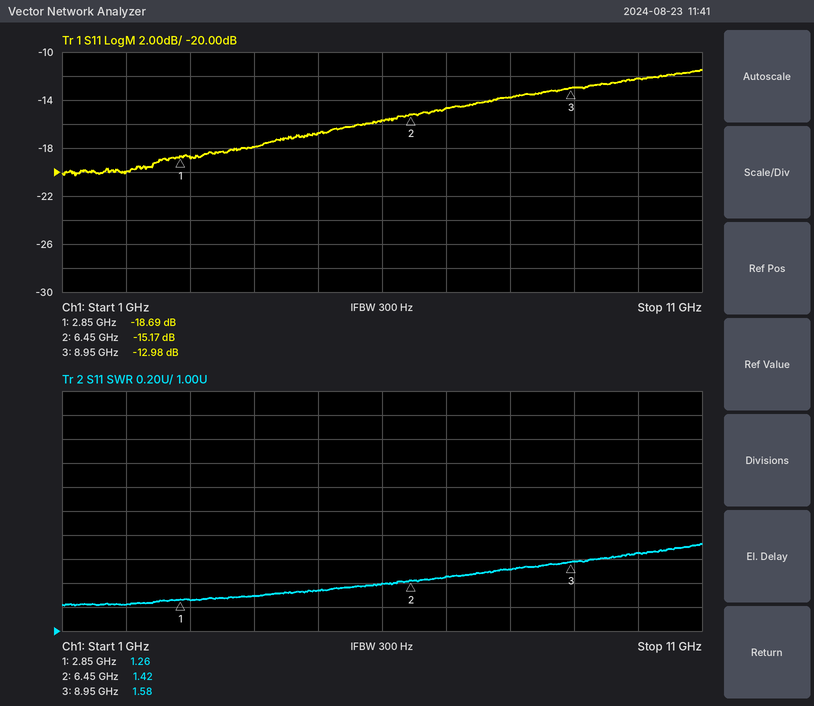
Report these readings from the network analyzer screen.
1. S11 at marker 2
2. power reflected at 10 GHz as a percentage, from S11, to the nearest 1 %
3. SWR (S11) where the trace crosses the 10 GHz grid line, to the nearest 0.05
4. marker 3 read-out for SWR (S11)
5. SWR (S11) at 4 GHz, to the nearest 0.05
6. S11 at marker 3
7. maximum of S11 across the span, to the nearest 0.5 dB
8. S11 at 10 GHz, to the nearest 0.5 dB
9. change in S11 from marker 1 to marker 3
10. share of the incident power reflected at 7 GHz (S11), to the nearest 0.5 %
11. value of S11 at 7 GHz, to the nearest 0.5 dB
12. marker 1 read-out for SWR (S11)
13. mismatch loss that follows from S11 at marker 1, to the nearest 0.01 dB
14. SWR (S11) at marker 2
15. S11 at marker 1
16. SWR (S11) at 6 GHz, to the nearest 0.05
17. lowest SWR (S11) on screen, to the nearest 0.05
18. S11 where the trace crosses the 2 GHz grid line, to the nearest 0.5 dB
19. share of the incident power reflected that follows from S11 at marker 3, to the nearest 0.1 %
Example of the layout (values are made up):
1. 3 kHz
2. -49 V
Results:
1. -15.17 dB
2. 6 %
3. 1.65
4. 1.58
5. 1.30
6. -12.98 dB
7. -11.5 dB
8. -12.0 dB
9. 5.71 dB
10. 3.5 %
11. -14.5 dB
12. 1.26
13. 0.06 dB
14. 1.42
15. -18.69 dB
16. 1.40
17. 1.20
18. -20.0 dB
19. 5.0 %
